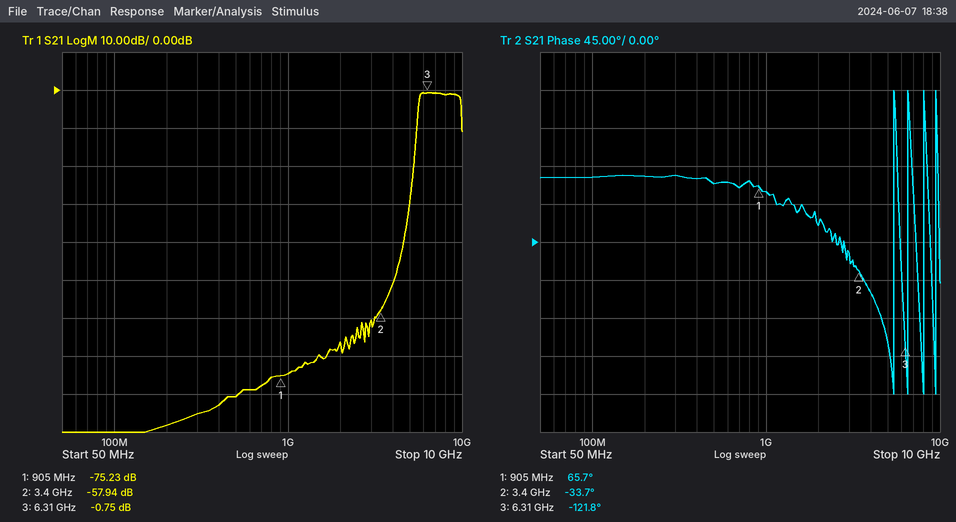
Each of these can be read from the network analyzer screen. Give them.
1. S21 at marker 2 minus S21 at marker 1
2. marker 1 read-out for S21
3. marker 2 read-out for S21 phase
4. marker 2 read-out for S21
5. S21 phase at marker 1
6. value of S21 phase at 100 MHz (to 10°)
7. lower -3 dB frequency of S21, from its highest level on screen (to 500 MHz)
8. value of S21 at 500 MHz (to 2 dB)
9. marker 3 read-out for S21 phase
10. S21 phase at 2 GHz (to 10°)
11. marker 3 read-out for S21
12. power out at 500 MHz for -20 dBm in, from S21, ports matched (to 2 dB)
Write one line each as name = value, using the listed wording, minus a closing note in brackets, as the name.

S21 at marker 2 minus S21 at marker 1 = 17.29 dB
marker 1 read-out for S21 = -75.23 dB
marker 2 read-out for S21 phase = -33.7°
marker 2 read-out for S21 = -57.94 dB
S21 phase at marker 1 = 65.7°
value of S21 phase at 100 MHz = 80°
lower -3 dB frequency of S21, from its highest level on screen = 5.5 GHz
value of S21 at 500 MHz = -80 dB
marker 3 read-out for S21 phase = -121.8°
S21 phase at 2 GHz = 20°
marker 3 read-out for S21 = -0.75 dB
power out at 500 MHz for -20 dBm in, from S21, ports matched = -100 dBm
